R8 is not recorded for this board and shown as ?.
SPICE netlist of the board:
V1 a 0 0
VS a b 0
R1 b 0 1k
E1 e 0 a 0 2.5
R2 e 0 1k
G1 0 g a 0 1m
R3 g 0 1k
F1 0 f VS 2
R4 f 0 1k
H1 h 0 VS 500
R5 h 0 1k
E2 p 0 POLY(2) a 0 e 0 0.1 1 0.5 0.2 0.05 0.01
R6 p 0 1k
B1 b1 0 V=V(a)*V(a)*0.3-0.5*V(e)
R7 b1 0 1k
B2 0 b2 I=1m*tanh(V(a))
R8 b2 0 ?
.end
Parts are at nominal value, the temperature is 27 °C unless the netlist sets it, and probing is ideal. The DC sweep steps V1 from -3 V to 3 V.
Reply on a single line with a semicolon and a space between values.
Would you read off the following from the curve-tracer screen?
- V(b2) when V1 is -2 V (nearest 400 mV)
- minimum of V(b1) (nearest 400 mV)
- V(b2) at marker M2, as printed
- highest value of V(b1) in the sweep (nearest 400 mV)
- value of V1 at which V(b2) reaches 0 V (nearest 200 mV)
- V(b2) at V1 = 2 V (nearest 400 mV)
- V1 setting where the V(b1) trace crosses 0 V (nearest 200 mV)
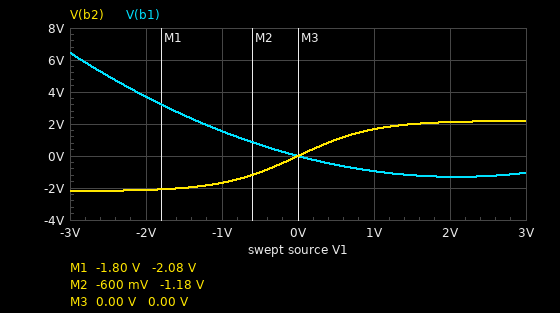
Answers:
-2.0 V; -1.2 V; -1.18 V; 6.4 V; 0 V; 2.0 V; 0 V
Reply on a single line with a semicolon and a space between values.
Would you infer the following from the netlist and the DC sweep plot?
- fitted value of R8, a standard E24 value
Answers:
2.2 kΩ
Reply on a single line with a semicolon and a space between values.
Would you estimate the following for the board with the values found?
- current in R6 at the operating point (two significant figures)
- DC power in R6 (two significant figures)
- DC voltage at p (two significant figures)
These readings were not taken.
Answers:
100 µA; 10 µW; 100 mV
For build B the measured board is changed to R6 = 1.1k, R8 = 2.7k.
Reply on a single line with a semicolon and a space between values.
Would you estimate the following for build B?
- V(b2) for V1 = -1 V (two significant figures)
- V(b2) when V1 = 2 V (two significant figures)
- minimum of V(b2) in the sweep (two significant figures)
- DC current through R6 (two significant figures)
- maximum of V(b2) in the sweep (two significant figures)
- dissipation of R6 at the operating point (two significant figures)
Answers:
-2.1 V; 2.6 V; -2.7 V; 91 µA; 2.7 V; 9.1 µW
